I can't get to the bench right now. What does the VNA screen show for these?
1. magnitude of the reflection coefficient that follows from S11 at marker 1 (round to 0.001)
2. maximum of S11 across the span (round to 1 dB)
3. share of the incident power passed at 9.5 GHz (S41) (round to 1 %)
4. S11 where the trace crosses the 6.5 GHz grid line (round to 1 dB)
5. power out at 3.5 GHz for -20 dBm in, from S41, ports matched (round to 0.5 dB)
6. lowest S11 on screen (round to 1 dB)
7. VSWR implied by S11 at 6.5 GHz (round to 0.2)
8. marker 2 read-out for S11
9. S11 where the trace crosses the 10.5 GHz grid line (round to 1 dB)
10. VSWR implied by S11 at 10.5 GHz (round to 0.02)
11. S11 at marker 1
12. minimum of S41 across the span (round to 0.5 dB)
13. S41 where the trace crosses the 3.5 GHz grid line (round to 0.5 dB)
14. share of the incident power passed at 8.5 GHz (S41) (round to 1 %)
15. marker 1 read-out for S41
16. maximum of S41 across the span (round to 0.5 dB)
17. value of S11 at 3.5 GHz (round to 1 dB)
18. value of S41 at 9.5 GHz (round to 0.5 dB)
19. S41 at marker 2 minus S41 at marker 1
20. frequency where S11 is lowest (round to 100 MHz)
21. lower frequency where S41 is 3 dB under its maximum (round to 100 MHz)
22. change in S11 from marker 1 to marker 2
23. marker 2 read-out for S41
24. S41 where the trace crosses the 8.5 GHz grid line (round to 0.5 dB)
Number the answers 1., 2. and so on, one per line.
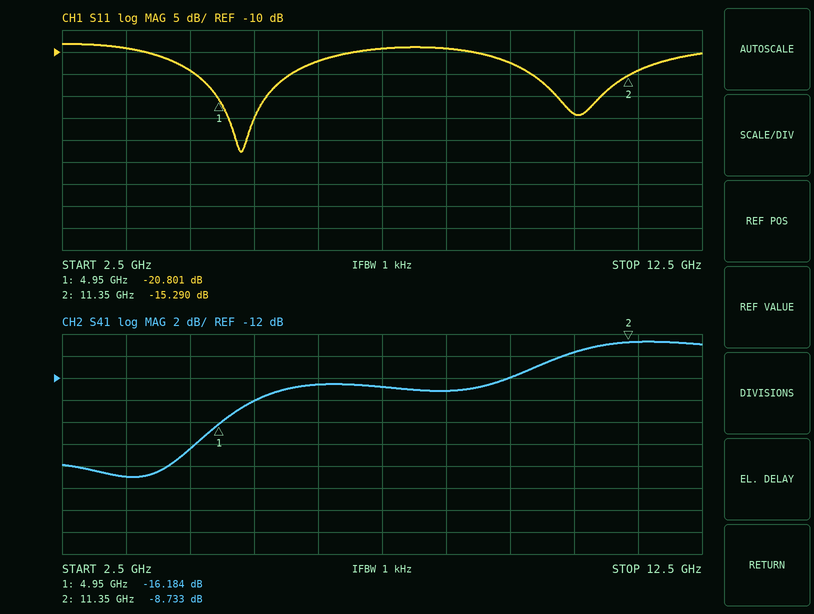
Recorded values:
1. 0.091
2. -8 dB
3. 6 %
4. -12 dB
5. -41.0 dBm
6. -33 dB
7. 1.6
8. -15.290 dB
9. -24 dB
10. 1.14
11. -20.801 dB
12. -21.0 dB
13. -21.0 dB
14. 5 %
15. -16.184 dB
16. -8.5 dB
17. -9 dB
18. -12.0 dB
19. 7.451 dB
20. 5.3 GHz
21. 9.6 GHz
22. 5.511 dB
23. -8.733 dB
24. -13.0 dB
